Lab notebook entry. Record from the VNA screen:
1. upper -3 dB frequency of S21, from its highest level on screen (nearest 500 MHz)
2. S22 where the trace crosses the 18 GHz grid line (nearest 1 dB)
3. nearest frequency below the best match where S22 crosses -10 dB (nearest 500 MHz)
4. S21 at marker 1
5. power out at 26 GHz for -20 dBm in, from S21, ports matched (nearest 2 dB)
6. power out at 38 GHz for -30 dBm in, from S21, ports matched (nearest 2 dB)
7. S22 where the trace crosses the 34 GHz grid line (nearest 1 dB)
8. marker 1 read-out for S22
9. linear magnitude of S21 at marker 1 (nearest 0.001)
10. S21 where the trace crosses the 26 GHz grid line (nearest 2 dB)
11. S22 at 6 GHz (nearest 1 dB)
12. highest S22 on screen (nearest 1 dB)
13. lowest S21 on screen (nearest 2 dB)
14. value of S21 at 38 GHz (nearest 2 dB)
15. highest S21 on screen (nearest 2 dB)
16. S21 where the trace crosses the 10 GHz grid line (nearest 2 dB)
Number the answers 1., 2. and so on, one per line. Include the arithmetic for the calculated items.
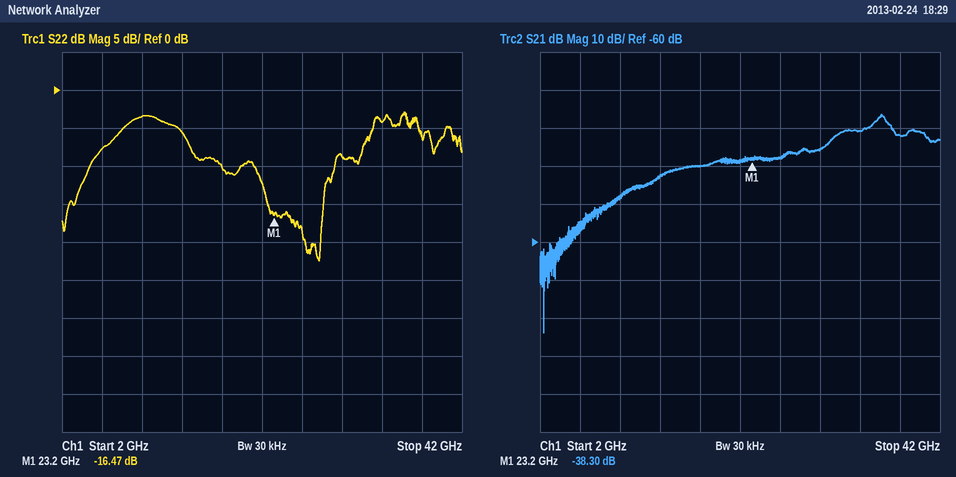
1. 37.0 GHz
2. -10 dB
3. 21.0 GHz
4. -38.30 dB
5. -20 dBm + (-38 dB) = -58 dBm
6. -30 dBm + (-32 dB) = -62 dBm
7. -4 dB
8. -16.47 dB
9. 10^(-38.3/20) ≈ 0.012
10. -38 dB
11. -8 dB
12. -3 dB
13. -84 dB
14. -32 dB
15. -26 dB
16. -48 dB
